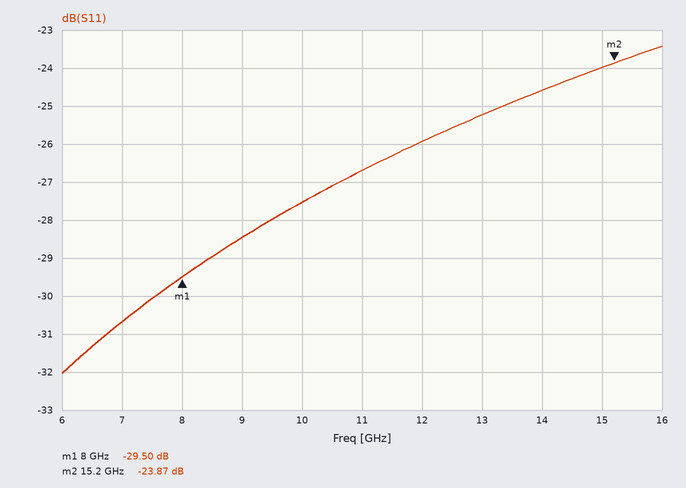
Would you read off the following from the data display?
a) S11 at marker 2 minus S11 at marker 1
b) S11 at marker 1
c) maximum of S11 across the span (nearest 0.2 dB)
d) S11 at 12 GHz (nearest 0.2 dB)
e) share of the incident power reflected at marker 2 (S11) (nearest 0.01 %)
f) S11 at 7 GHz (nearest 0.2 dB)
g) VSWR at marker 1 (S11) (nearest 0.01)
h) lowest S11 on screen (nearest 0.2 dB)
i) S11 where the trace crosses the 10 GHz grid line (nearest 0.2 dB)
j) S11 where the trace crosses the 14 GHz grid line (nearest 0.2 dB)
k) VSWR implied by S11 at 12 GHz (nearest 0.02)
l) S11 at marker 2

5.63 dB
-29.50 dB
-23.4 dB
-26.0 dB
0.41 %
-30.6 dB
1.07
-32.0 dB
-27.6 dB
-24.6 dB
1.10
-23.87 dB
